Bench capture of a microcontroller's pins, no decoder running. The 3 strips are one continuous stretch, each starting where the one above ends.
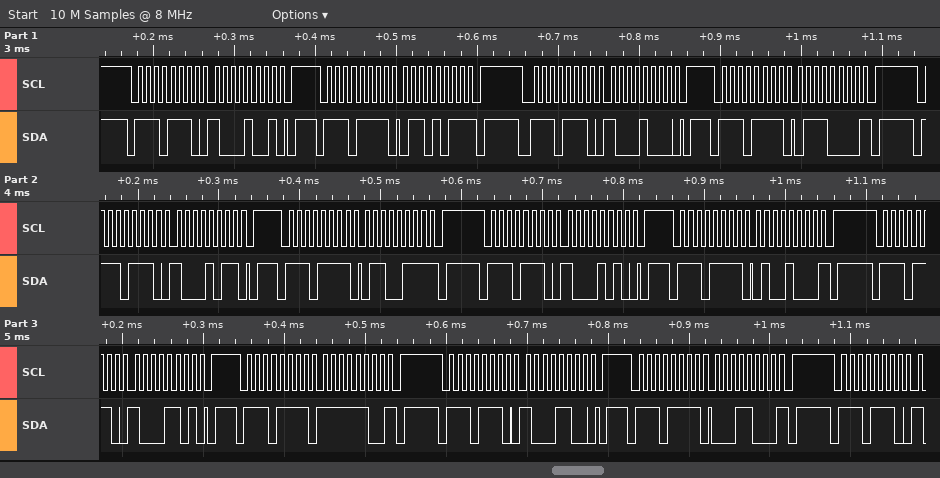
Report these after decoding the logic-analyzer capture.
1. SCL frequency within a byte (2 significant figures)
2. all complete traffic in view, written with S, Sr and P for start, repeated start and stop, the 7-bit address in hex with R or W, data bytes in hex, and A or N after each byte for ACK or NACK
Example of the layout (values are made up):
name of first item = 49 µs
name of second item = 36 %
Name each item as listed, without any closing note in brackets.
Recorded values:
SCL frequency within a byte = 100 kHz
all complete traffic in view, written with S, Sr and P for start, repeated start and stop, the 7-bit address in hex with R or W, data bytes in hex, and A or N after each byte for ACK or NACK = S 77W A 89 A P S 77R A 6B N P S 77W A 88 A P S 77R A 70 N P S 77W A 8B A P S 77R A 67 N P S 77W A 8A A P S 77R A 48 N P S 77W A 8D A P S 77R A FC N P S 77W A 8C A P S 77R A 18 N P S 77W A
